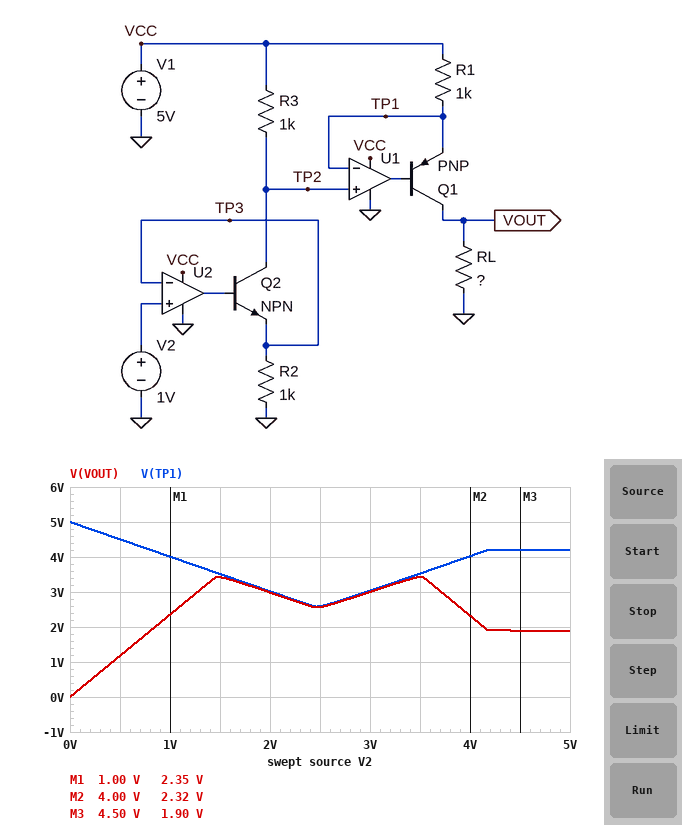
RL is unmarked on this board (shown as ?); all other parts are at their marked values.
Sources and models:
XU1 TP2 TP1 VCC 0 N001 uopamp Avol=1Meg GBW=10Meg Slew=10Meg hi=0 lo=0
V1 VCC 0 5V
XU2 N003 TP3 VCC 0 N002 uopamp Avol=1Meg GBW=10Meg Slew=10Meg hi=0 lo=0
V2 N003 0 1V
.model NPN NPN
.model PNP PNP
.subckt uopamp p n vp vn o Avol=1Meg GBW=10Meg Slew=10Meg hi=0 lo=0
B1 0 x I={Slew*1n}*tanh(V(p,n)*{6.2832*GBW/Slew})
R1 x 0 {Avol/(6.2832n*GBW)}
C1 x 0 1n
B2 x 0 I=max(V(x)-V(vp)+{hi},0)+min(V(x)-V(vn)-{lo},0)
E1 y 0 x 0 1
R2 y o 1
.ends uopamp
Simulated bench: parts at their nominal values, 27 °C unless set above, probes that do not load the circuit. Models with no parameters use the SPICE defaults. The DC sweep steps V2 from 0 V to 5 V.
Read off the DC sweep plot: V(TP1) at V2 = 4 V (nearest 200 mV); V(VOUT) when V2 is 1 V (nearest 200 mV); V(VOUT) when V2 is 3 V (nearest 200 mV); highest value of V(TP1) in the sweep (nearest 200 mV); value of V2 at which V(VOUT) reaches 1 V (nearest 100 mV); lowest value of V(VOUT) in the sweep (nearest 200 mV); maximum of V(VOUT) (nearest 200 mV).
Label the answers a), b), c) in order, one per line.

a) 4.0 V
b) 2.4 V
c) 3.0 V
d) 5.0 V
e) 400 mV
f) 0 V
g) 3.4 V
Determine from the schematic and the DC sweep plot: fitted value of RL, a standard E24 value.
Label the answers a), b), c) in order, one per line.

a) 2.4 kΩ
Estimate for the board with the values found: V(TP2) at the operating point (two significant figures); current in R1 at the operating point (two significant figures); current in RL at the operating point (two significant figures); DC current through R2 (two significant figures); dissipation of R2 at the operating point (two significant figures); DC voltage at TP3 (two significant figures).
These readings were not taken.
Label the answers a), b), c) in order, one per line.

a) 4.0 V
b) 990 µA
c) 980 µA
d) 1.0 mA
e) 1.0 mW
f) 1.0 V
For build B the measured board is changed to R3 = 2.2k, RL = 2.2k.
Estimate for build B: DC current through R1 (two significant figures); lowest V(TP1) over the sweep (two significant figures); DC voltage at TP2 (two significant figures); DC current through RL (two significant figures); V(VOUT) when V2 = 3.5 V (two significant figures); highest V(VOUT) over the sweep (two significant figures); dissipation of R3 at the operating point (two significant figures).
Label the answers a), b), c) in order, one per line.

a) 2.2 mA
b) 1.7 V
c) 2.8 V
d) 1.3 mA
e) 3.2 V
f) 3.3 V
g) 2.2 mW
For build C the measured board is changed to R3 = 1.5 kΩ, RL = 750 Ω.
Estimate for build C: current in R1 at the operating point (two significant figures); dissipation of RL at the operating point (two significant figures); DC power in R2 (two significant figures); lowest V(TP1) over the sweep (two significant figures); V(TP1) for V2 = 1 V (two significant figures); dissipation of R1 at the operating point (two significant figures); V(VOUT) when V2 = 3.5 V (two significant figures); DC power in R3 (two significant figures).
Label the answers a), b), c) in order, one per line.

a) 1.5 mA
b) 1.6 mW
c) 1.0 mW
d) 2.1 V
e) 3.5 V
f) 2.2 mW
g) 1.1 V
h) 1.5 mW
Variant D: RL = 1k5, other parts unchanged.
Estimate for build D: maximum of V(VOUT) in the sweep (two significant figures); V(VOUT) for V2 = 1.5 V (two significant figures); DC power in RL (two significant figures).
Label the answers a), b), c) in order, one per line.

a) 2.9 V
b) 2.2 V
c) 1.4 mW
